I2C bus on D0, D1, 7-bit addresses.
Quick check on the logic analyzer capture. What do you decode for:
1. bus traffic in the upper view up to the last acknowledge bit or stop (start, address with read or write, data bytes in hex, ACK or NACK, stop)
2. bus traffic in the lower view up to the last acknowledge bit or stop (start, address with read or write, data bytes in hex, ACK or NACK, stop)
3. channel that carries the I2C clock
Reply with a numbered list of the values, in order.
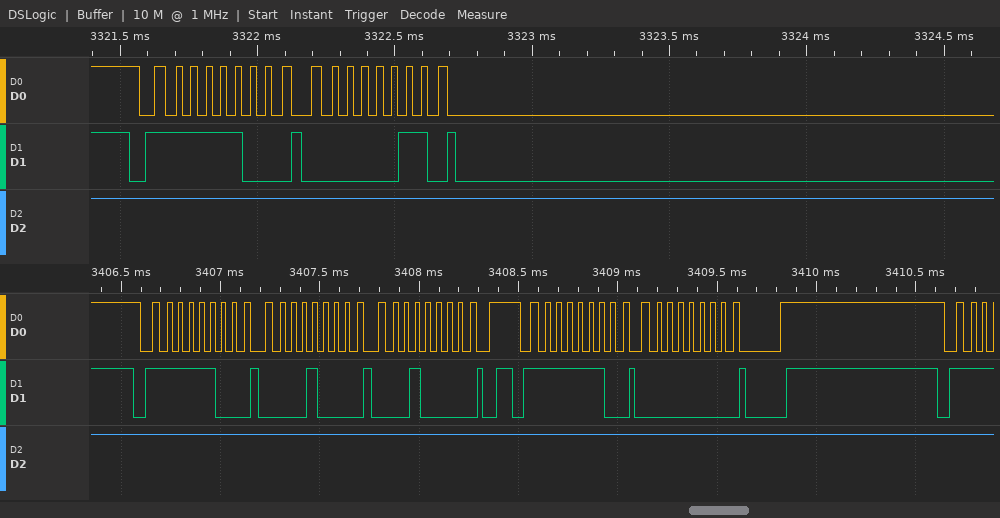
1. start, address 7E write ACK, 03 ACK
2. start, address 7E write ACK, 08 ACK, 10 ACK, stop, start, address 7F write ACK, 00 ACK, stop
3. D0
